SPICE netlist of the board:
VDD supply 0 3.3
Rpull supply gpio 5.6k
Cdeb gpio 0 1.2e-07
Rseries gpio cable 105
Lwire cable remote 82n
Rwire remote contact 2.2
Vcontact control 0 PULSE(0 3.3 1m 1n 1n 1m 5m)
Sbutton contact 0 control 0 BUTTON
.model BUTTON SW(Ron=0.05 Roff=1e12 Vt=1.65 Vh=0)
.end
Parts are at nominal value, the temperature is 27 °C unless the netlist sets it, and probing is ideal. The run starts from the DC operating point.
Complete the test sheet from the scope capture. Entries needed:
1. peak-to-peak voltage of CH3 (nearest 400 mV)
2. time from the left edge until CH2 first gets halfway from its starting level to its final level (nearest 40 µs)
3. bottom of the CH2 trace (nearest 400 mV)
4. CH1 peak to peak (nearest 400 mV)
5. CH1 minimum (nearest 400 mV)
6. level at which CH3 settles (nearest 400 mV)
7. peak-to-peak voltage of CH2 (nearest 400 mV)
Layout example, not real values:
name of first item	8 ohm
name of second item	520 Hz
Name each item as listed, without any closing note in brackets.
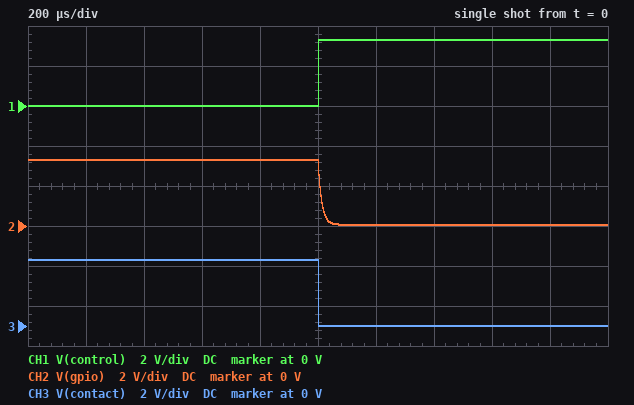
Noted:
peak-to-peak voltage of CH3	3.2 V
time from the left edge until CH2 first gets halfway from its starting level to its final level	1.00 ms
bottom of the CH2 trace	0 V
CH1 peak to peak	3.2 V
CH1 minimum	0 V
level at which CH3 settles	0 V
peak-to-peak voltage of CH2	3.2 V
